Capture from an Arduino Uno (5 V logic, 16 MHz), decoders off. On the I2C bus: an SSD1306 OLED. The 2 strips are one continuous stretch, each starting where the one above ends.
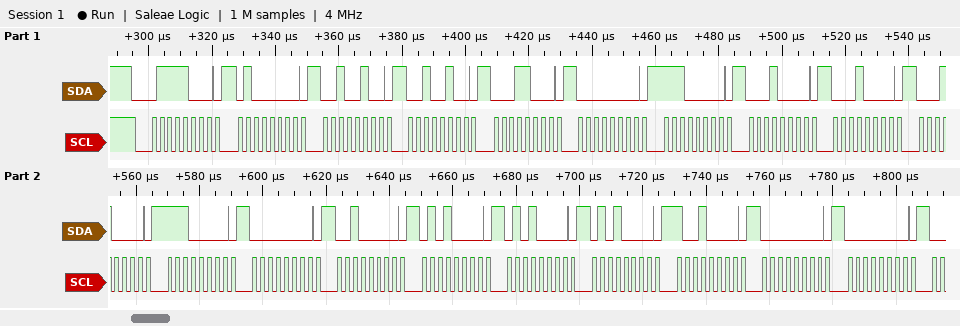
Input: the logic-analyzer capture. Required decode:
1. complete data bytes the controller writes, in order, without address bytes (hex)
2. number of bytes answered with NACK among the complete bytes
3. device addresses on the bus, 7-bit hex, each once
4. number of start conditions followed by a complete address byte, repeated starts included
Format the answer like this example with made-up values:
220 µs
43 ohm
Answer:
40 24 24 18 00 E0 10 10 10 E0 00 20 50 50 50 90 00 00
0
0x3C
1
